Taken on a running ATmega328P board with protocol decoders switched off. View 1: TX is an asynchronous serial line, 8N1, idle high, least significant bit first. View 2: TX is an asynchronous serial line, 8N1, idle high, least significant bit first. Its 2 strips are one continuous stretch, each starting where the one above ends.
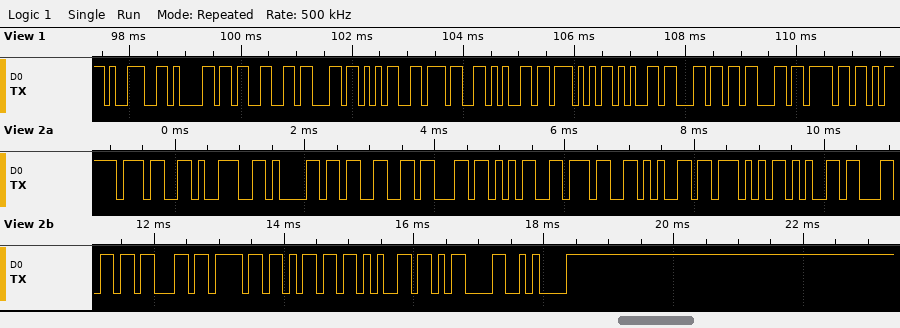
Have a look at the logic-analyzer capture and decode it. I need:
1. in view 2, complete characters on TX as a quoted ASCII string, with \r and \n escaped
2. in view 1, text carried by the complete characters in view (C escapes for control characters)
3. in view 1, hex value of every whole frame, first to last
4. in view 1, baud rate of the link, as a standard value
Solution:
"79a3c57eWelcome\r\n"
"9a3c57eWelco"
0x39 0x61 0x33 0x63 0x35 0x37 0x65 0x57 0x65 0x6C 0x63 0x6F
9600 baud
